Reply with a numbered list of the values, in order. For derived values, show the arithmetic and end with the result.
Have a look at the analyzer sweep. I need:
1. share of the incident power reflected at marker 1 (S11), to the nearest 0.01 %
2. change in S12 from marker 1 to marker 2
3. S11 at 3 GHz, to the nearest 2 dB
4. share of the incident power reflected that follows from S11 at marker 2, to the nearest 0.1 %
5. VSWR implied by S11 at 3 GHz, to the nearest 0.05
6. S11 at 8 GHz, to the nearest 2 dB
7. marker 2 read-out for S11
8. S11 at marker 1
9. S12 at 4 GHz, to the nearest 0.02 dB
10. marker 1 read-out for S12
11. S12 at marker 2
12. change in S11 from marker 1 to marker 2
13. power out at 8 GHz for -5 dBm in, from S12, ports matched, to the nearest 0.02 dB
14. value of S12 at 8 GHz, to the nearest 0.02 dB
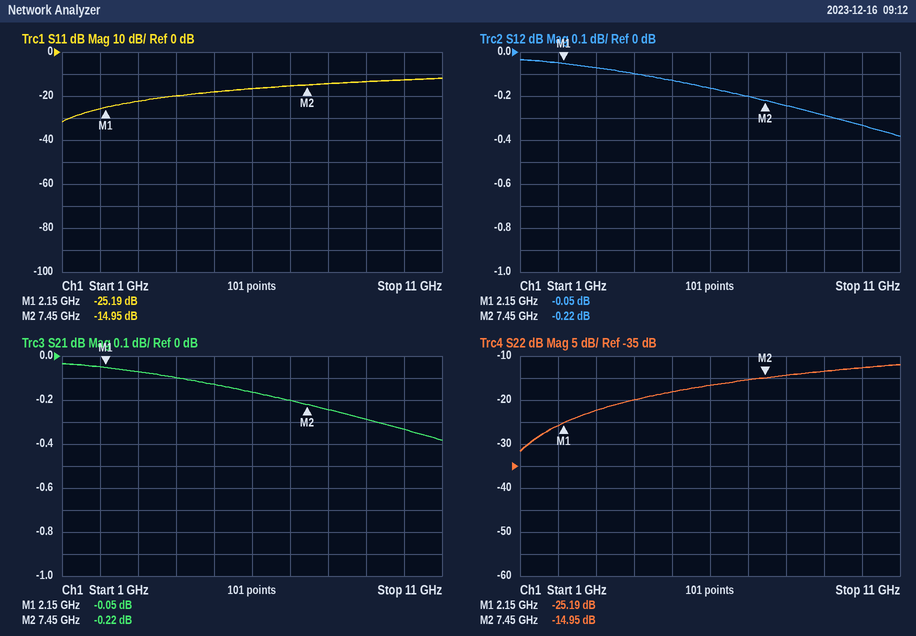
1. 10^(-25.19/10) ≈ 0.30 %
2. -0.22 − (-0.05) = -0.17 dB
3. -22 dB
4. 10^(-14.95/10) ≈ 3.2 %
5. |Γ| = 10^(-22/20) = 0.0794; VSWR = (1 + 0.0794)/(1 − 0.0794) ≈ 1.17, so 1.15 to the nearest 0.05
6. -14 dB
7. -14.95 dB
8. -25.19 dB
9. -0.10 dB
10. -0.05 dB
11. -0.22 dB
12. -14.95 − (-25.19) = 10.24 dB
13. -5 dBm + (-0.24 dB) = -5.24 dBm
14. -0.24 dB
